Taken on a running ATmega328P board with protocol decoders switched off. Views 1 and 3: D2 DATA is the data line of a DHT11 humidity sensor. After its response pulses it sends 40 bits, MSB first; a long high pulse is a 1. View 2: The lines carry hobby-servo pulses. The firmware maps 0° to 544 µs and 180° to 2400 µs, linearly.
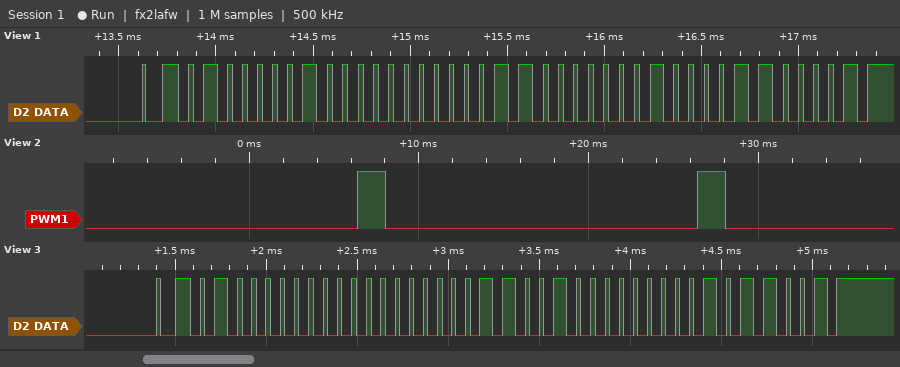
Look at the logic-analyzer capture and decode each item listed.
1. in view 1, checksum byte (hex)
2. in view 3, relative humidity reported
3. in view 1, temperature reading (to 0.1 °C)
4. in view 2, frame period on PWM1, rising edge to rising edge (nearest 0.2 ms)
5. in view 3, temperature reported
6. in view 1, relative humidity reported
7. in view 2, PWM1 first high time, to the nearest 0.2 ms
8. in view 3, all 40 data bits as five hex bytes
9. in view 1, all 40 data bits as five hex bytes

0x61
64 %
24.8 °C
20.0 ms
25.0 °C
65 %
1.6 ms
40 00 19 00 59
41 00 18 08 61
